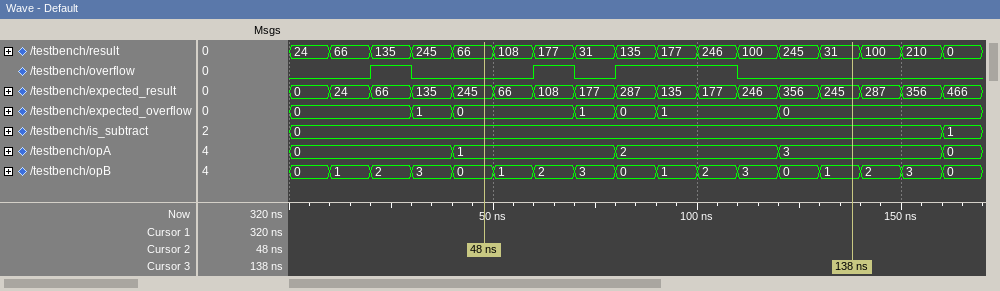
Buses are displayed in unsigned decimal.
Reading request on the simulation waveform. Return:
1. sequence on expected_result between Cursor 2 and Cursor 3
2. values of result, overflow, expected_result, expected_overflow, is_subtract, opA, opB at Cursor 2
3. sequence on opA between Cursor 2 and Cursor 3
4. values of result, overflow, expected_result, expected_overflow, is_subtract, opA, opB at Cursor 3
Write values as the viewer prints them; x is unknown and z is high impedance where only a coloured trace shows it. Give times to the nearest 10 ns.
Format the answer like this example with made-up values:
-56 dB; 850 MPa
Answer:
245, 66, 108, 177, 287, 135, 177, 246, 356, 245; result=66, overflow=0, expected_result=245, expected_overflow=0, is_subtract=0, opA=1, opB=0; 1, 2, 3; result=31, overflow=0, expected_result=245, expected_overflow=0, is_subtract=0, opA=3, opB=1
